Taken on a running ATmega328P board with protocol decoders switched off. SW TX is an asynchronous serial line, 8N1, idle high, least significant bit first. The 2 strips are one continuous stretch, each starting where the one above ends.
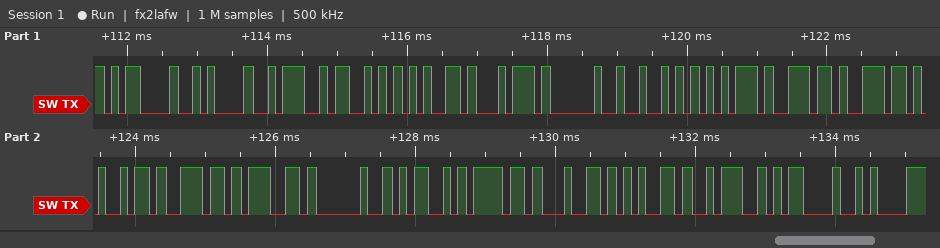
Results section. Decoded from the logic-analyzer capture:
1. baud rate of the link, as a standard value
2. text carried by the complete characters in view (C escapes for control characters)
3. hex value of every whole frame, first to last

9600 baud
"\r\n:Set Running Mode:\r\n"
0x0D 0x0A 0x3A 0x53 0x65 0x74 0x20 0x52 0x75 0x6E 0x6E 0x69 0x6E 0x67 0x20 0x4D 0x6F 0x64 0x65 0x3A 0x0D 0x0A
